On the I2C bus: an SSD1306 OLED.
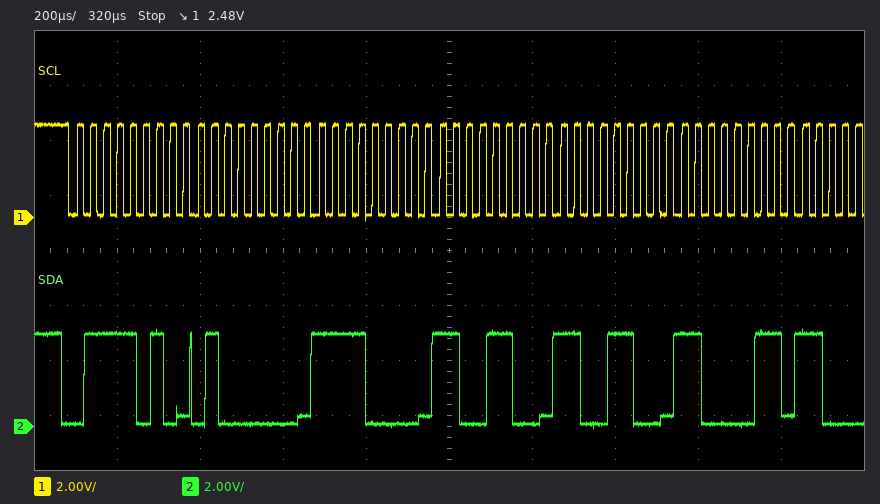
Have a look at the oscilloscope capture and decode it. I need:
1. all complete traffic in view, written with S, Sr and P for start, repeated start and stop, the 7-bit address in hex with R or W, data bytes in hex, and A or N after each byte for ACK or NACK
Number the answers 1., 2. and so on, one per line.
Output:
1. S 3DW A 40 A F0 A CC A CC A C3 A
